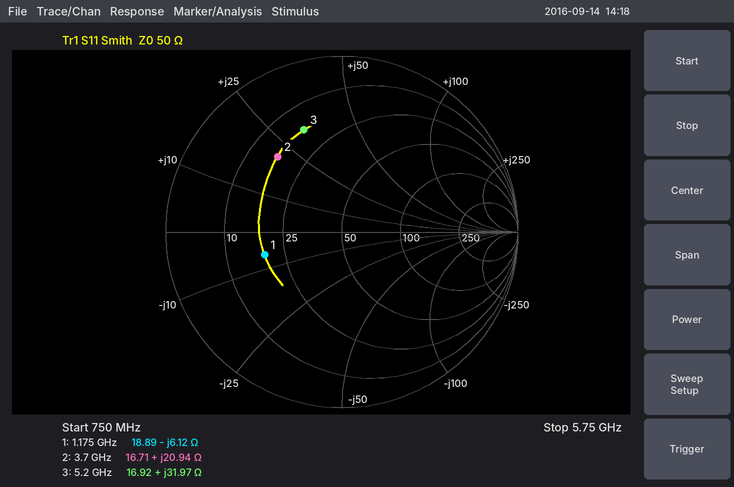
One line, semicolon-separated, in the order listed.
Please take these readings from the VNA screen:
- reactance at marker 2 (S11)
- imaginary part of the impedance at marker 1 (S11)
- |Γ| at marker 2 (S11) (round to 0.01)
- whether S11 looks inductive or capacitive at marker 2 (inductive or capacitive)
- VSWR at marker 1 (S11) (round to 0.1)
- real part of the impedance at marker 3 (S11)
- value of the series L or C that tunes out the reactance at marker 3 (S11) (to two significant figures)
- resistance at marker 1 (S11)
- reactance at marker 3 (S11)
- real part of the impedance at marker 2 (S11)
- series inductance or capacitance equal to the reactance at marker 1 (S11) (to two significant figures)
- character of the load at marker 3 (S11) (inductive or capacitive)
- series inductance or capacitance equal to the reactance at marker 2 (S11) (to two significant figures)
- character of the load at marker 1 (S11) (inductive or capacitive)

+20.94 Ω; -6.12 Ω; 0.56; inductive; 2.7; 16.92 Ω; 960 fF; 18.89 Ω; +31.97 Ω; 16.71 Ω; 22 pF; inductive; 900 pH; capacitive
